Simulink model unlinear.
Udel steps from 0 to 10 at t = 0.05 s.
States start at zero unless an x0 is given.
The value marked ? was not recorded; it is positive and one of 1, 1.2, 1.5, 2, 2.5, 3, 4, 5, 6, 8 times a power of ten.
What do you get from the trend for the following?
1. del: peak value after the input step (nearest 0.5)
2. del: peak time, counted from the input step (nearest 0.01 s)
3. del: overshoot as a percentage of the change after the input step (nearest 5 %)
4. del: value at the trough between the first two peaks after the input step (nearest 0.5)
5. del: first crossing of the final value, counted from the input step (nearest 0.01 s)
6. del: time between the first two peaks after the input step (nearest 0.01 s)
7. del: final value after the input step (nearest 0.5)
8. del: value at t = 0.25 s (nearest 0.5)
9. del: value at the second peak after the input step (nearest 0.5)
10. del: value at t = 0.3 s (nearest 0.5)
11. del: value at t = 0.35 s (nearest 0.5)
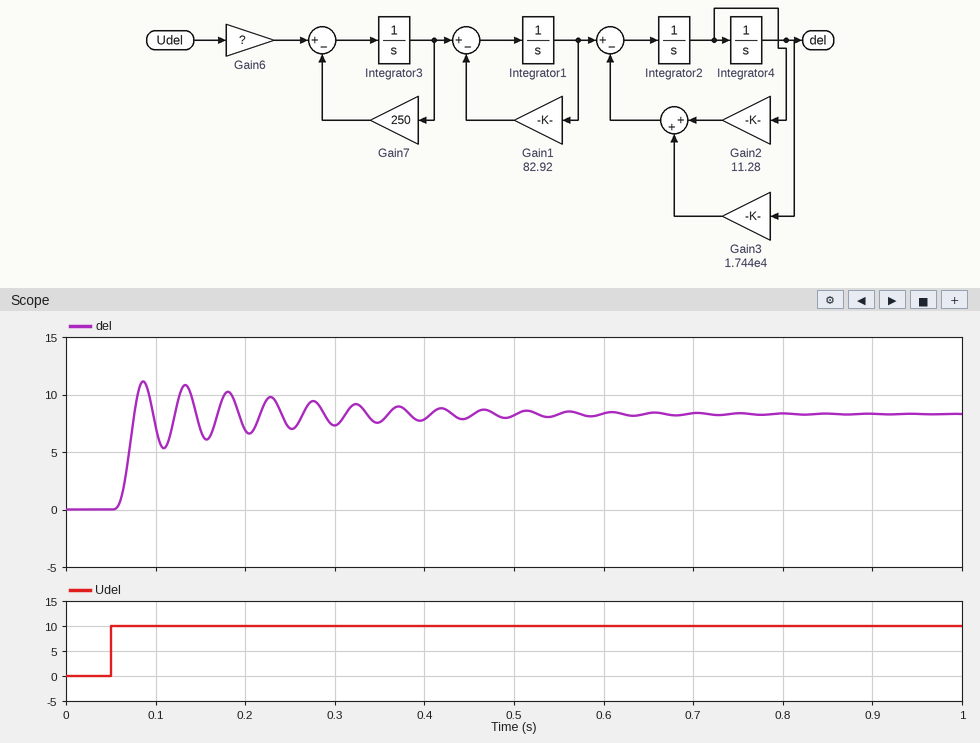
11.0
0.04 s
35 %
5.5
0.03 s
0.05 s
8.5
7.0
11.0
7.5
7.5
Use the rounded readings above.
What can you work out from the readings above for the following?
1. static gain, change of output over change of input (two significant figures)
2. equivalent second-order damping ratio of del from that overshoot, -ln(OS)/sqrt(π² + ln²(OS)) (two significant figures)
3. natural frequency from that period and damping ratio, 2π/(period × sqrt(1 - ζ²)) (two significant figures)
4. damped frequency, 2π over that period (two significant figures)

0.85
0.32
130 rad/s
130 rad/s
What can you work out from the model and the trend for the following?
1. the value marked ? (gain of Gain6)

3e+08
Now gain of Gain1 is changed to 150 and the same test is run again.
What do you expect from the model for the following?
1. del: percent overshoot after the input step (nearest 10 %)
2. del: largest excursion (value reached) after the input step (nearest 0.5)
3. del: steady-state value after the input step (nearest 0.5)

60 %
7.0
4.5
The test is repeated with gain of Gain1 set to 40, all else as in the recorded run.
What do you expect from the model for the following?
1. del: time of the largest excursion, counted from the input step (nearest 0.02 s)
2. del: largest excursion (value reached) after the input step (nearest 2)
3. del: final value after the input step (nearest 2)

0.08 s
20
18
